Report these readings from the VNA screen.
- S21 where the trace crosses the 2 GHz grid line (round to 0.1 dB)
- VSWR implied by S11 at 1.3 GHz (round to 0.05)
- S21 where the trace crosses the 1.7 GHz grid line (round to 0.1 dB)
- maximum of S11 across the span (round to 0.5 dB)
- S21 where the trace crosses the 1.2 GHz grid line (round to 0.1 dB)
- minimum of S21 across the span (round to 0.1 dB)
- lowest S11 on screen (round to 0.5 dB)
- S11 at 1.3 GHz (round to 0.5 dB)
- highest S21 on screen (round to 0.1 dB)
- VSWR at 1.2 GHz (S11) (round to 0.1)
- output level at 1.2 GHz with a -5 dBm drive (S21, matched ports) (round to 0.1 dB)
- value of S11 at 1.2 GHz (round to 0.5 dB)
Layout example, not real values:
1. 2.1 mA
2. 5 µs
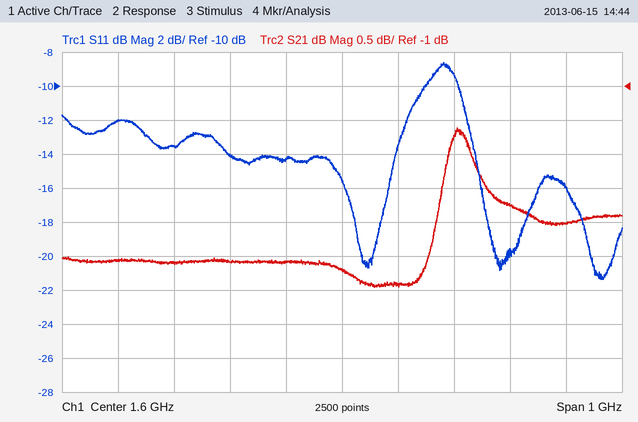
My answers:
1. -3.0 dB
2. 1.55
3. -3.9 dB
4. -8.5 dB
5. -3.6 dB
6. -4.0 dB
7. -21.5 dB
8. -13.5 dB
9. -1.6 dB
10. 1.7
11. -8.6 dBm
12. -12.0 dB
